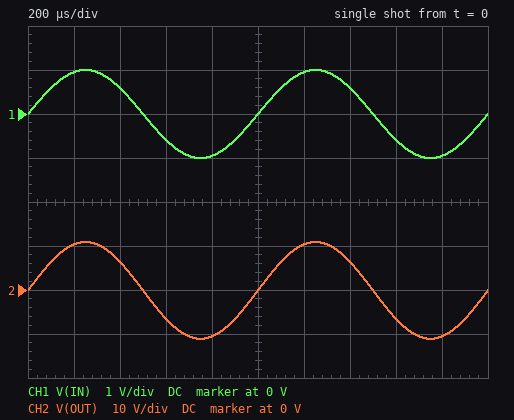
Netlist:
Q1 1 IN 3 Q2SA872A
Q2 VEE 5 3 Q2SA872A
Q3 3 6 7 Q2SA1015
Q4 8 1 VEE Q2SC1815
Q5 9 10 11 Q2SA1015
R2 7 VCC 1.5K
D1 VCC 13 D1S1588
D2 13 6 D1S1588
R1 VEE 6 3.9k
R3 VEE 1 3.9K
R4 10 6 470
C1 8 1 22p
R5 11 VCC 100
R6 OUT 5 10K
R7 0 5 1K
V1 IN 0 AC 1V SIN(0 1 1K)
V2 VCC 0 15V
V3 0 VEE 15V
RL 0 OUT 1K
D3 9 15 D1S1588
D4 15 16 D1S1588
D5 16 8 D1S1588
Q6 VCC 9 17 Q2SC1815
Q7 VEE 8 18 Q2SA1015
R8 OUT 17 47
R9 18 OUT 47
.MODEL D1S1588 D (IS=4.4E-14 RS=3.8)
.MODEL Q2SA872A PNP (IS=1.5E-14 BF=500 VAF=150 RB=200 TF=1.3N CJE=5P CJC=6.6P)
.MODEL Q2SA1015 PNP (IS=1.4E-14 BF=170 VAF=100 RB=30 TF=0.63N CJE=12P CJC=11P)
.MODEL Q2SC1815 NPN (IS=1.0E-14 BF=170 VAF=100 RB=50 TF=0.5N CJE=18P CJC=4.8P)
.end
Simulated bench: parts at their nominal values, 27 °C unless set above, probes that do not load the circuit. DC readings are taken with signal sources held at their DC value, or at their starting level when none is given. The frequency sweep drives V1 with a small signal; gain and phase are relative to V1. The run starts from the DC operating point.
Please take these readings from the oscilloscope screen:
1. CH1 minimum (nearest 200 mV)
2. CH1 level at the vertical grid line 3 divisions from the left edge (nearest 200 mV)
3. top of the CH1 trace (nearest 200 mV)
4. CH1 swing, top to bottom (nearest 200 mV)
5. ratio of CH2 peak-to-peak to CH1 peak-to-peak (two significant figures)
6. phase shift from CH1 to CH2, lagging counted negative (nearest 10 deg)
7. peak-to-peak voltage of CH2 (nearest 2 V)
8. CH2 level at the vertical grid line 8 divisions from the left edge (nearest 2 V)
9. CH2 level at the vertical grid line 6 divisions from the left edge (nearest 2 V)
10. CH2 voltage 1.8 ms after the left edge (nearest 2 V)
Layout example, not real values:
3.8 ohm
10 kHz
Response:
-1.0 V
-600 mV
1.0 V
2.0 V
11
0 deg
22 V
-6 V
10 V
-10 V
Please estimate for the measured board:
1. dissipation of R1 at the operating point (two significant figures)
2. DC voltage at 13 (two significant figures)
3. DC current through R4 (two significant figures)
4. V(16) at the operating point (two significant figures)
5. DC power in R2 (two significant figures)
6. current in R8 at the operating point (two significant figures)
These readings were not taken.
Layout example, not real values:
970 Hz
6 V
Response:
210 mW
14 V
35 µA
-430 mV
390 µW
7.1 mA
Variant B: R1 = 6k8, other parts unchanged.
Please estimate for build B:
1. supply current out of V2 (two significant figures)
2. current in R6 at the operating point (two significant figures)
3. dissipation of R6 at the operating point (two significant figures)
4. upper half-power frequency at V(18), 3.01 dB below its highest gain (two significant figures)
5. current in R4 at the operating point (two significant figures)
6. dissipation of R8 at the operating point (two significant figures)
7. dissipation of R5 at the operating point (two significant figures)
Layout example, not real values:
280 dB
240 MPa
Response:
18 mA
5.7 µA
330 nW
3.6 MHz
33 µA
2.3 mW
4.0 mW
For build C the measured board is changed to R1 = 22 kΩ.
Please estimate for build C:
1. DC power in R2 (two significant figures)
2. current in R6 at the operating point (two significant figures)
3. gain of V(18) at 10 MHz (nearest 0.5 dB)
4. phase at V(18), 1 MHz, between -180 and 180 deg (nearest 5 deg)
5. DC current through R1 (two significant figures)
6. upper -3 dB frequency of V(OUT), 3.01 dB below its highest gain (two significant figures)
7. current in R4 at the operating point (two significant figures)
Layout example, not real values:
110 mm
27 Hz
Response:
270 µW
950 nA
7.0 dB
-25 deg
1.3 mA
3.1 MHz
29 µA
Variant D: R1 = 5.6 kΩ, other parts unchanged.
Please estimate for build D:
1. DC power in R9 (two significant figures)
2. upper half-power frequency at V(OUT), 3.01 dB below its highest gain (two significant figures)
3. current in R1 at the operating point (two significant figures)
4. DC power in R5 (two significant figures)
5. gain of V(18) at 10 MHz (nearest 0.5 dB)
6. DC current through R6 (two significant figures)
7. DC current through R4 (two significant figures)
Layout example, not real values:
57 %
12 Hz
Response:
2.4 mW
3.6 MHz
5.1 mA
4.2 mW
8.0 dB
6.6 µA
34 µA
